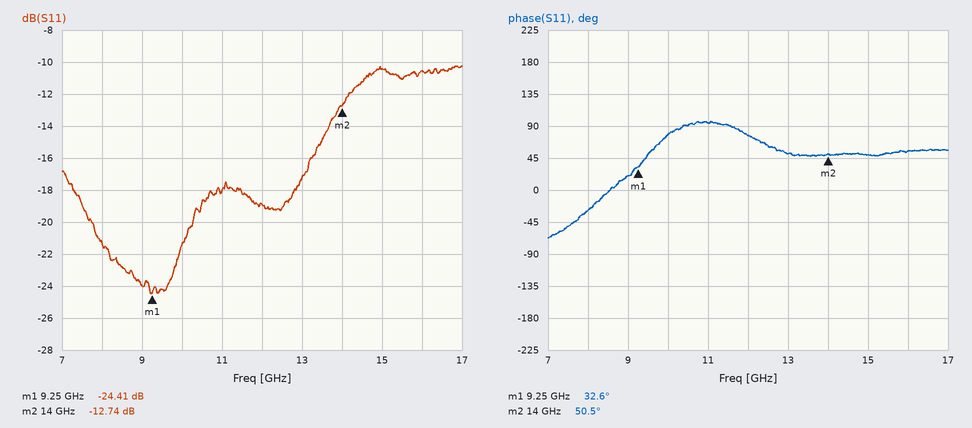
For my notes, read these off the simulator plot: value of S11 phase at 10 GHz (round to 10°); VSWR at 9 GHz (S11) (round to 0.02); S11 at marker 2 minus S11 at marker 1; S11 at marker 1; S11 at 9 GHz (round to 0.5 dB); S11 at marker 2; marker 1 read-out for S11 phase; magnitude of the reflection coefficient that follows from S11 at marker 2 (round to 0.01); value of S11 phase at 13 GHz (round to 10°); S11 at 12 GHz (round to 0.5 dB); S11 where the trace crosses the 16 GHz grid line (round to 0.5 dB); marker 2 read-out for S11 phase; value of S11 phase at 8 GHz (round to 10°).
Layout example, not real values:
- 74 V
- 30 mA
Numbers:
- 80°
- 1.14
- 11.67 dB
- -24.41 dB
- -24.0 dB
- -12.74 dB
- 32.6°
- 0.23
- 50°
- -19.0 dB
- -10.5 dB
- 50.5°
- -30°
